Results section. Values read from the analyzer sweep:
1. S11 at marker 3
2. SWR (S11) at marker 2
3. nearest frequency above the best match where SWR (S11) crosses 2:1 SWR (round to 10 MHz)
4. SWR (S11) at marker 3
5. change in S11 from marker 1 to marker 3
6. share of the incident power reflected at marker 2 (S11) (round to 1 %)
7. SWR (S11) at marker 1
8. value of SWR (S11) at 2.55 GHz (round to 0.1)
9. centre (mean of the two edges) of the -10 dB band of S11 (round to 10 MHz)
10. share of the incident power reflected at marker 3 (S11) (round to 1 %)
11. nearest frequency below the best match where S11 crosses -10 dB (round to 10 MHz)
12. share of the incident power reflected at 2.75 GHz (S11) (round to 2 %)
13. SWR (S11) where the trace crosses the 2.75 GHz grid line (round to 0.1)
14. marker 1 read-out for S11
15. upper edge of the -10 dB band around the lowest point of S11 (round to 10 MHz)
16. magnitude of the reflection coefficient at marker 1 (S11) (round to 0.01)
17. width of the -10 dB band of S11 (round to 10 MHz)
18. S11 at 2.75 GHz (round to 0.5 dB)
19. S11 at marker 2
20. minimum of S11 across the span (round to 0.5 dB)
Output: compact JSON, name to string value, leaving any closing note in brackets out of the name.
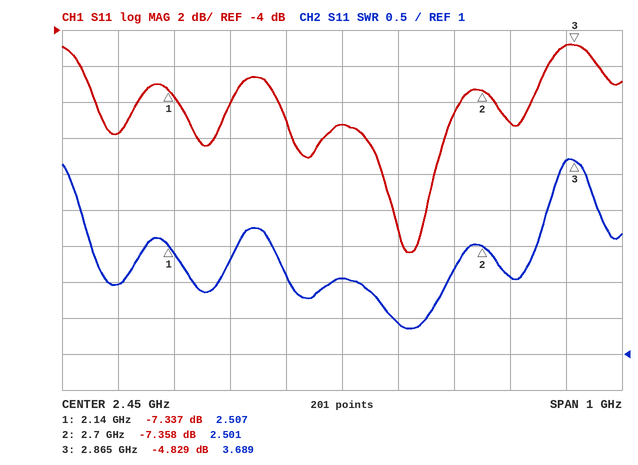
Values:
{"S11 at marker 3": "-4.829 dB", "SWR (S11) at marker 2": "2.501", "nearest frequency above the best match where SWR (S11) crosses 2:1 SWR": "2.64 GHz", "SWR (S11) at marker 3": "3.689", "change in S11 from marker 1 to marker 3": "2.508 dB", "share of the incident power reflected at marker 2 (S11)": "18 %", "SWR (S11) at marker 1": "2.507", "value of SWR (S11) at 2.55 GHz": "1.4", "centre (mean of the two edges) of the -10 dB band of S11": "2.56 GHz", "share of the incident power reflected at marker 3 (S11)": "33 %", "nearest frequency below the best match where S11 crosses -10 dB": "2.49 GHz", "share of the incident power reflected at 2.75 GHz (S11)": "12 %", "SWR (S11) where the trace crosses the 2.75 GHz grid line": "2.1", "marker 1 read-out for S11": "-7.337 dB", "upper edge of the -10 dB band around the lowest point of S11": "2.63 GHz", "magnitude of the reflection coefficient at marker 1 (S11)": "0.43", "width of the -10 dB band of S11": "140 MHz", "S11 at 2.75 GHz": "-9.0 dB", "S11 at marker 2": "-7.358 dB", "minimum of S11 across the span": "-16.5 dB"}
